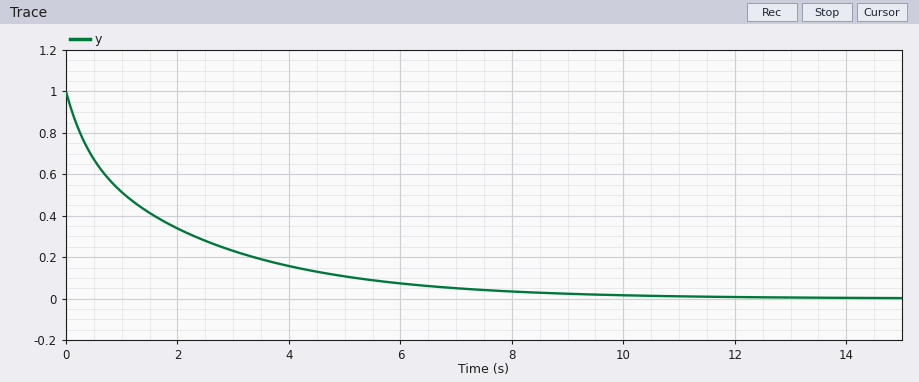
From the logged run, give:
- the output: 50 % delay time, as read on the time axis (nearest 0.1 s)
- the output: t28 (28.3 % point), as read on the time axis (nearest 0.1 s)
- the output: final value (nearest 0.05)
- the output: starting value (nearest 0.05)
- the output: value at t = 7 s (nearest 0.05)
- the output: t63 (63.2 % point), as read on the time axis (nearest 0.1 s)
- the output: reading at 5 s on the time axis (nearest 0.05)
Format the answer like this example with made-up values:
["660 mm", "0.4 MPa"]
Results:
["1.1 s", "0.4 s", "0.00", "1.00", "0.05", "1.8 s", "0.10"]
